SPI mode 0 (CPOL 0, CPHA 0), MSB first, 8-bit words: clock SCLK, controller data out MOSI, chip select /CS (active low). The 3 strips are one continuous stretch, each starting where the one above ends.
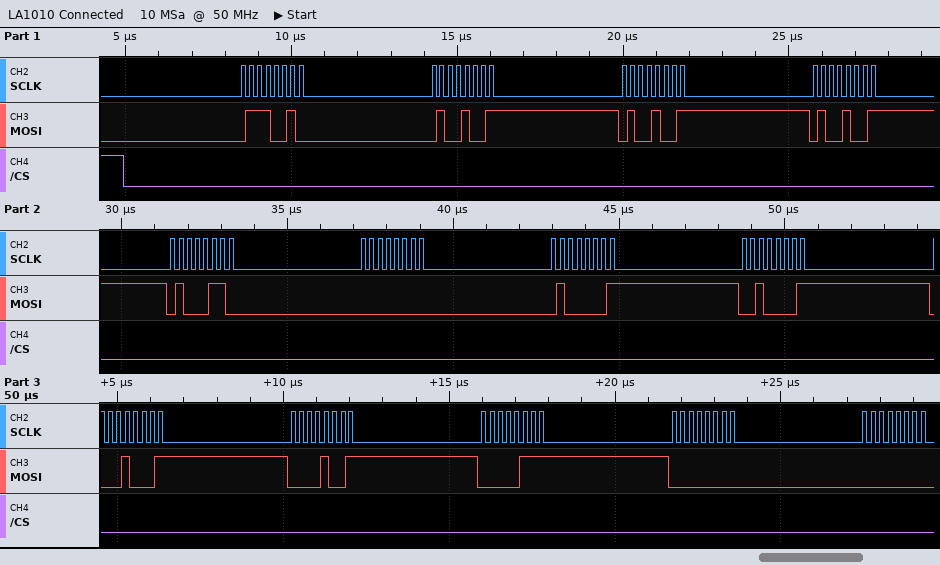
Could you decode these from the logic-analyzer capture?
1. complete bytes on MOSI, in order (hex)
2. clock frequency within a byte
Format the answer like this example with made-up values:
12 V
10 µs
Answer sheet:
72 49 49 49 46 00 41 21 11 09 07 00 00
4 MHz
